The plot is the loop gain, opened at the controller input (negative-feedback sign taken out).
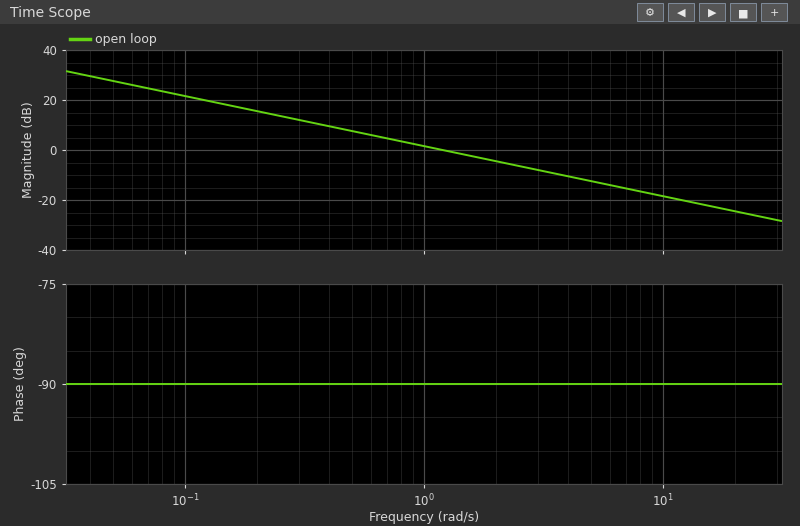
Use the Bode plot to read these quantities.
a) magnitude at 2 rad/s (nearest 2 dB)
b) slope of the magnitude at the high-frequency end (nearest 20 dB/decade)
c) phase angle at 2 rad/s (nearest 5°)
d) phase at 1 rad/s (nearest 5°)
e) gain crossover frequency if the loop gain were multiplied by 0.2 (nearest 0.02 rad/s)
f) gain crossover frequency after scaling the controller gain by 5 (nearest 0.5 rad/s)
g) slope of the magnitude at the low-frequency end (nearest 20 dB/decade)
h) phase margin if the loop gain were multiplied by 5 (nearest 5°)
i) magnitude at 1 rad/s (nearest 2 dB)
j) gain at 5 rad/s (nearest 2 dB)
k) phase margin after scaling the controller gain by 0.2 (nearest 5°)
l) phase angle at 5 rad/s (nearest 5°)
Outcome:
-4 dB
-20 dB/decade
-90°
-90°
0.24 rad/s
6.0 rad/s
-20 dB/decade
90°
2 dB
-12 dB
90°
-90°
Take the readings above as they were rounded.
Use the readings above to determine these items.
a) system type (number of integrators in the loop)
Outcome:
1
